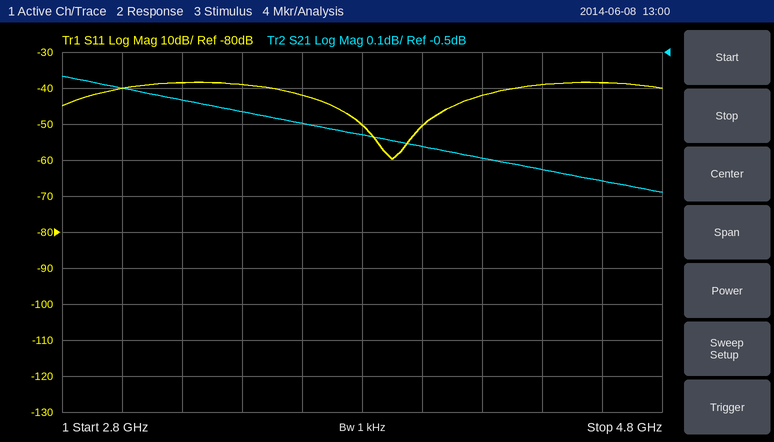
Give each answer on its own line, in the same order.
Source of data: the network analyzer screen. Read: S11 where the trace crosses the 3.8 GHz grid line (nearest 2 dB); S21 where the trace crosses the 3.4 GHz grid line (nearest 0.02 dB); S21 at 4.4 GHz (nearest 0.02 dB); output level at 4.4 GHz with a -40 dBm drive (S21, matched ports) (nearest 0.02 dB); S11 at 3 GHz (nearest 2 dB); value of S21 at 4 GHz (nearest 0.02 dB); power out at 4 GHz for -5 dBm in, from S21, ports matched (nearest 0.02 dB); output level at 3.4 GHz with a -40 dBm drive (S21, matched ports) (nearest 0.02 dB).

-50 dB
-0.66 dB
-0.82 dB
-40.82 dBm
-40 dB
-0.76 dB
-5.76 dBm
-40.66 dBm
